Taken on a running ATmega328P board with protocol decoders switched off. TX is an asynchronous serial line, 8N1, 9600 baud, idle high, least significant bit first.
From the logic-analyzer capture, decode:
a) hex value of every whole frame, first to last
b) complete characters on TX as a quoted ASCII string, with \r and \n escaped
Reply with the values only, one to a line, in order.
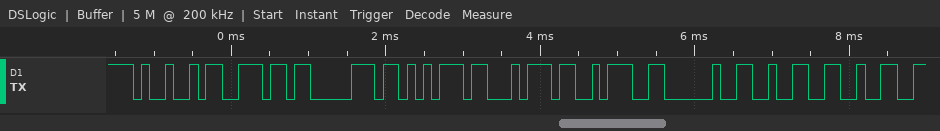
0x49 0x6E 0x70 0x75 0x74 0x3A 0x20 0x32 0x32
"Input: 22"
